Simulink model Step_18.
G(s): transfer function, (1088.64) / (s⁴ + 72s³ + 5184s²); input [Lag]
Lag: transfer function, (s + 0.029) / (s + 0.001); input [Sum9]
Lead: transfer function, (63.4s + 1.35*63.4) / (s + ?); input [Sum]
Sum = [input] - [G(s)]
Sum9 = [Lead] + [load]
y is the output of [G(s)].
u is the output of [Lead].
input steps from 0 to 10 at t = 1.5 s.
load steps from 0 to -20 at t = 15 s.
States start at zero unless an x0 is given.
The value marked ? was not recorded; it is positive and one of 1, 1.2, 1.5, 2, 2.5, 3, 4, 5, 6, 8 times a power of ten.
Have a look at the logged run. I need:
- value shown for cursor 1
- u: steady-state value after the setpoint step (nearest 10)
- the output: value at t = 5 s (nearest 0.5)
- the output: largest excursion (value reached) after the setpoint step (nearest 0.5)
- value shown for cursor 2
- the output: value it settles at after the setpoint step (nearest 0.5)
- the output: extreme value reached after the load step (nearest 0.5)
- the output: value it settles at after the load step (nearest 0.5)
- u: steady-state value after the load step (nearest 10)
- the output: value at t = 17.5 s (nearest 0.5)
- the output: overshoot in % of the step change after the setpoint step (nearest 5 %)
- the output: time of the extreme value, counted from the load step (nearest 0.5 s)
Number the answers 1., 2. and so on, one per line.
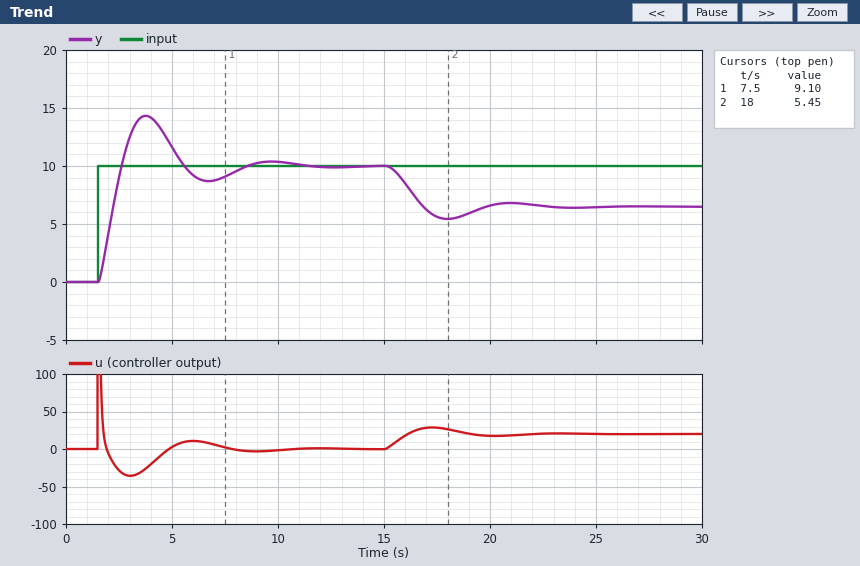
1. 9.10
2. 0
3. 11.5
4. 14.5
5. 5.45
6. 10.0
7. 5.5
8. 6.5
9. 20
10. 5.5
11. 45 %
12. 3.0 s
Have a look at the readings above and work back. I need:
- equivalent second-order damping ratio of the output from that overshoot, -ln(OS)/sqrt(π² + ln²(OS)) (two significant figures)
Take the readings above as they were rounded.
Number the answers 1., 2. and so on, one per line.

1. 0.25
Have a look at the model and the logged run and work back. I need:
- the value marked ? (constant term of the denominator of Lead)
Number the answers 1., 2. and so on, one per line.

1. 15
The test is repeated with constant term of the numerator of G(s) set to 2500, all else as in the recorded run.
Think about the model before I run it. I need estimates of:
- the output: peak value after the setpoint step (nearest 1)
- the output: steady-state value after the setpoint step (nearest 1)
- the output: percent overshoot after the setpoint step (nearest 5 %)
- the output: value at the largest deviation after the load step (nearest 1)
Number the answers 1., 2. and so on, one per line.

1. 13
2. 10
3. 30 %
4. 6
